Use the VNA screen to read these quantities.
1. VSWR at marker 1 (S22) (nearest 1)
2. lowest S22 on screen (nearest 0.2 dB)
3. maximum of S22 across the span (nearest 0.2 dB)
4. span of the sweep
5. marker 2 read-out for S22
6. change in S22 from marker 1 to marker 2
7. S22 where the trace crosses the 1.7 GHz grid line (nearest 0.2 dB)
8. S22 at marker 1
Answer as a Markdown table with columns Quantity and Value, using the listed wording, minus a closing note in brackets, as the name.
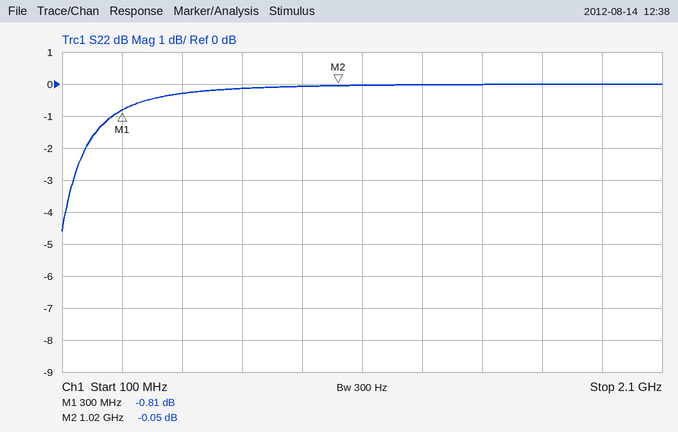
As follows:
| Quantity | Value |
|---|---|
| VSWR at marker 1 (S22) | 21 |
| lowest S22 on screen | -4.6 dB |
| maximum of S22 across the span | 0.0 dB |
| span of the sweep | 2 GHz |
| marker 2 read-out for S22 | -0.05 dB |
| change in S22 from marker 1 to marker 2 | 0.76 dB |
| S22 where the trace crosses the 1.7 GHz grid line | 0.0 dB |
| S22 at marker 1 | -0.81 dB |
